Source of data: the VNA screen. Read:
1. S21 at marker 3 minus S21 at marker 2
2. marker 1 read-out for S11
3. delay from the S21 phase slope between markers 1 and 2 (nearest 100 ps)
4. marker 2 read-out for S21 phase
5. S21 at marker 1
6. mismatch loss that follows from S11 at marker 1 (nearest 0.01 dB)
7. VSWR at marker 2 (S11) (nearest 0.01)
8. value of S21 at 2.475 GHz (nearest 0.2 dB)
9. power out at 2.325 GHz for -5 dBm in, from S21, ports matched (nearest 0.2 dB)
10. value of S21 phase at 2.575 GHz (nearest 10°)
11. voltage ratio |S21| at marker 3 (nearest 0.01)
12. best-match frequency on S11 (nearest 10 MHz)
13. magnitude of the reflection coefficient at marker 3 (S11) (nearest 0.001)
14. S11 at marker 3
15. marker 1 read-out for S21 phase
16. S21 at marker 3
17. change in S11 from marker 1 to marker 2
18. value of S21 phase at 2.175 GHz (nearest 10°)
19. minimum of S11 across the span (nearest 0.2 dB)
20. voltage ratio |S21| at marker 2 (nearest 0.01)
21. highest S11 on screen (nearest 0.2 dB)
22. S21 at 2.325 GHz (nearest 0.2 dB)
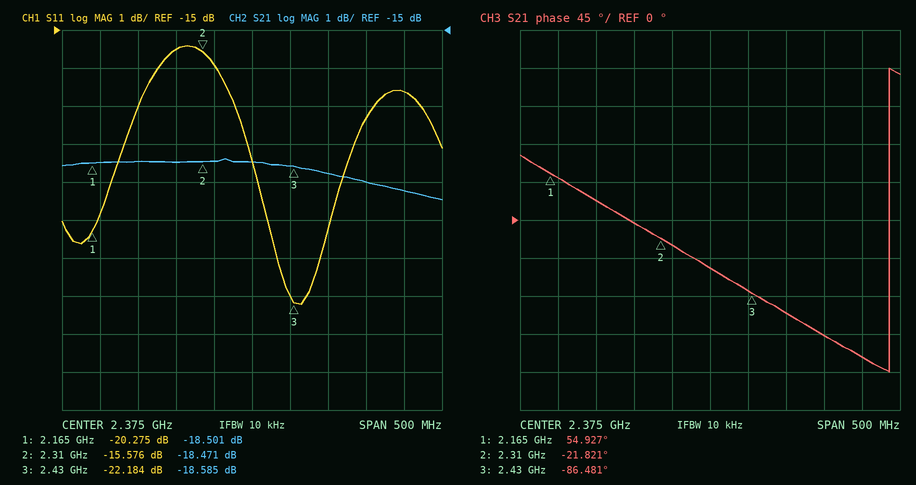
-0.114 dB
-20.275 dB
1.5 ns
-21.821°
-18.501 dB
0.04 dB
1.40
-18.8 dB
-23.4 dBm
-160°
0.12
2.44 GHz
0.078
-22.184 dB
54.927°
-18.585 dB
4.699 dB
50°
-22.2 dB
0.12
-15.4 dB
-18.4 dB
